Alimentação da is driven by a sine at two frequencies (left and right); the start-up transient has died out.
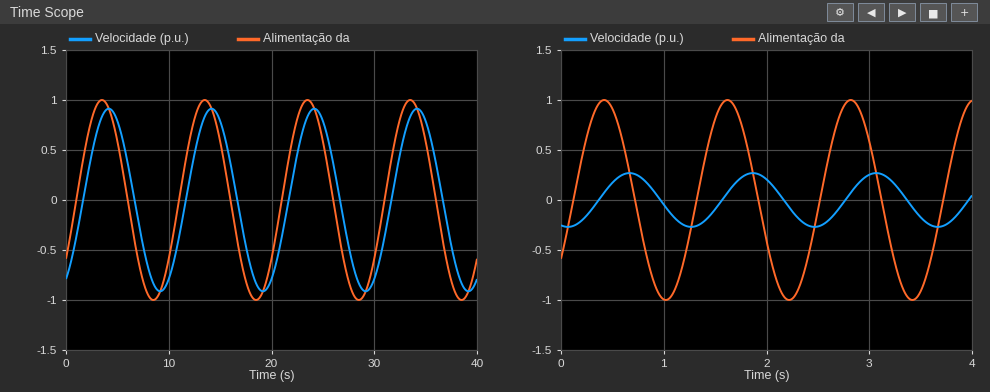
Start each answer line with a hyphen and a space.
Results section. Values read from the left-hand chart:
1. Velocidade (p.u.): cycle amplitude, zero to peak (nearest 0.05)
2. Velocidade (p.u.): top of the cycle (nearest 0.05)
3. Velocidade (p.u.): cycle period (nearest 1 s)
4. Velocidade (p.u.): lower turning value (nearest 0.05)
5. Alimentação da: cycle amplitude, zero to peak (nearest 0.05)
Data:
- 0.90
- 0.90
- 10 s
- -0.90
- 1.00
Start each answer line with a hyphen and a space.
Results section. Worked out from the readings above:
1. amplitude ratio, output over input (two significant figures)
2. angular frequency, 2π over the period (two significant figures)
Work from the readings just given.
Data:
- 0.90
- 0.63 rad/s
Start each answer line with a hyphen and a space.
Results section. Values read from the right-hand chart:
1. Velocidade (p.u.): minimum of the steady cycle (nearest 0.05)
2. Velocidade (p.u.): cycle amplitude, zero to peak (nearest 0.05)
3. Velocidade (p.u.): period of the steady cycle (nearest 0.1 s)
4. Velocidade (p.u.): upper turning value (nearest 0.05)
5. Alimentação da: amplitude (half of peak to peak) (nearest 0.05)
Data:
- -0.25
- 0.25
- 1.2 s
- 0.25
- 1.00
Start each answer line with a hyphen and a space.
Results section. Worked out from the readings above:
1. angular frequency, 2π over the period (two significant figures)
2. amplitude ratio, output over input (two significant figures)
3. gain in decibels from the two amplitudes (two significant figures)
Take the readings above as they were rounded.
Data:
- 5.2 rad/s
- 0.25
- -12 dB
